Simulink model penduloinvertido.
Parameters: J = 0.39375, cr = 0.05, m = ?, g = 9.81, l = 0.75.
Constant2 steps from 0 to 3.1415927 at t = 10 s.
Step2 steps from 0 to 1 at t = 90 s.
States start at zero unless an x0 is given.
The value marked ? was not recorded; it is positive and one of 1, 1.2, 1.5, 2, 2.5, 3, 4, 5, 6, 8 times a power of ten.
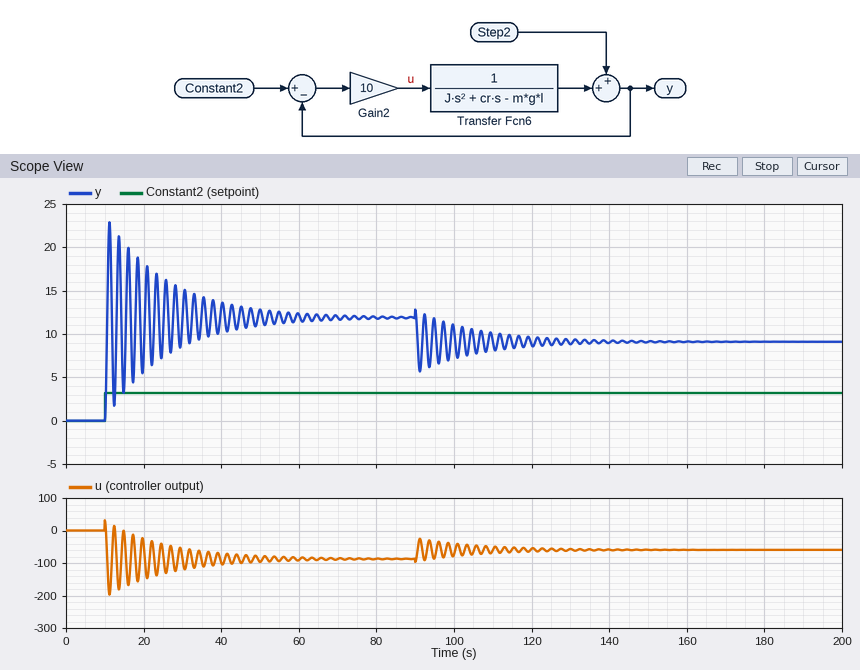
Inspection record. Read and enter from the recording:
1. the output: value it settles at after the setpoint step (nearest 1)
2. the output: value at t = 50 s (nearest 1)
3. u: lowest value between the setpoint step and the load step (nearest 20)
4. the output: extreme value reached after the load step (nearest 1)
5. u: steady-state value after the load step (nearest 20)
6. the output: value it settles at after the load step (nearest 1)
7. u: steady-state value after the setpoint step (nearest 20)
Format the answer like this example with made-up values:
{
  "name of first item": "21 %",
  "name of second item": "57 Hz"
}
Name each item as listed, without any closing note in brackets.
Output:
{
  "the output: value it settles at after the setpoint step": "12",
  "the output: value at t = 50 s": "13",
  "u: lowest value between the setpoint step and the load step": "-200",
  "the output: extreme value reached after the load step": "6",
  "u: steady-state value after the load step": "-60",
  "the output: value it settles at after the load step": "9",
  "u: steady-state value after the setpoint step": "-80"
}
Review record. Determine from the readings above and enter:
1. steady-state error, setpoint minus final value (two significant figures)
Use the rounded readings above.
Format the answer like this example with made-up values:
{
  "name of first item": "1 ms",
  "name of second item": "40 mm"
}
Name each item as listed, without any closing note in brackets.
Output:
{
  "steady-state error, setpoint minus final value": "-8.9"
}
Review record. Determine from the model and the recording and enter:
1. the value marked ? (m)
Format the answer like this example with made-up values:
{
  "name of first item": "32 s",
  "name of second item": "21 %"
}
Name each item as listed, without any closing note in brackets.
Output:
{
  "the value marked ?": "1"
}
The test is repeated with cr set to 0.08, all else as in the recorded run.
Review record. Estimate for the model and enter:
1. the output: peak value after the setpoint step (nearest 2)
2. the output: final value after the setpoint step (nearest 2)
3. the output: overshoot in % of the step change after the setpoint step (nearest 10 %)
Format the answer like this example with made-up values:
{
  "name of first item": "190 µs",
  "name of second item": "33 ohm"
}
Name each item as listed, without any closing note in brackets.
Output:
{
  "the output: peak value after the setpoint step": "22",
  "the output: final value after the setpoint step": "12",
  "the output: overshoot in % of the step change after the setpoint step": "90 %"
}
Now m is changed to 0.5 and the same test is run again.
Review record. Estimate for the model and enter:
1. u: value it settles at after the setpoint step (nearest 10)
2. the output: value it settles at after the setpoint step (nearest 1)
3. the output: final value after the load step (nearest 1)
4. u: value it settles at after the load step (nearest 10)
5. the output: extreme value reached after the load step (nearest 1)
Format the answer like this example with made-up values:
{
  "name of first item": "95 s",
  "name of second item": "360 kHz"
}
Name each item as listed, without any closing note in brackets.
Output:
{
  "u: value it settles at after the setpoint step": "-20",
  "the output: value it settles at after the setpoint step": "5",
  "the output: final value after the load step": "4",
  "u: value it settles at after the load step": "-10",
  "the output: extreme value reached after the load step": "3"
}
